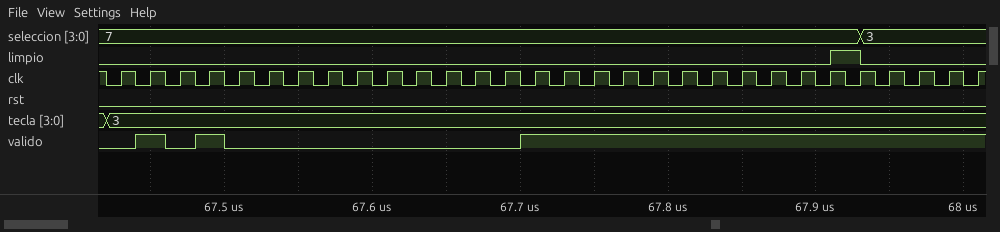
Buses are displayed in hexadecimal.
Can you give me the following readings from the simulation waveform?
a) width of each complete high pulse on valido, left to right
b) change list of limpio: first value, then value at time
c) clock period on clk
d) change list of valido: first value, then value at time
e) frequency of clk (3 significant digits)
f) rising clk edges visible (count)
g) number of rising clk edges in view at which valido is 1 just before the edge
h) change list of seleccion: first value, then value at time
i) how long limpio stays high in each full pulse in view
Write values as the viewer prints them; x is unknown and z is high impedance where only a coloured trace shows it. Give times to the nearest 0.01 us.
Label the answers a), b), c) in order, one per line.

a) 0.02 us, 0.02 us
b) 0, 1 at 67.91 us, 0 at 67.93 us
c) 0.02 us
d) 0, 1 at 67.44 us, 0 at 67.46 us, 1 at 67.48 us, 0 at 67.5 us, 1 at 67.7 us
e) 50.0 MHz
f) 30
g) 18
h) 7, 3 at 67.93 us
i) 0.02 us
